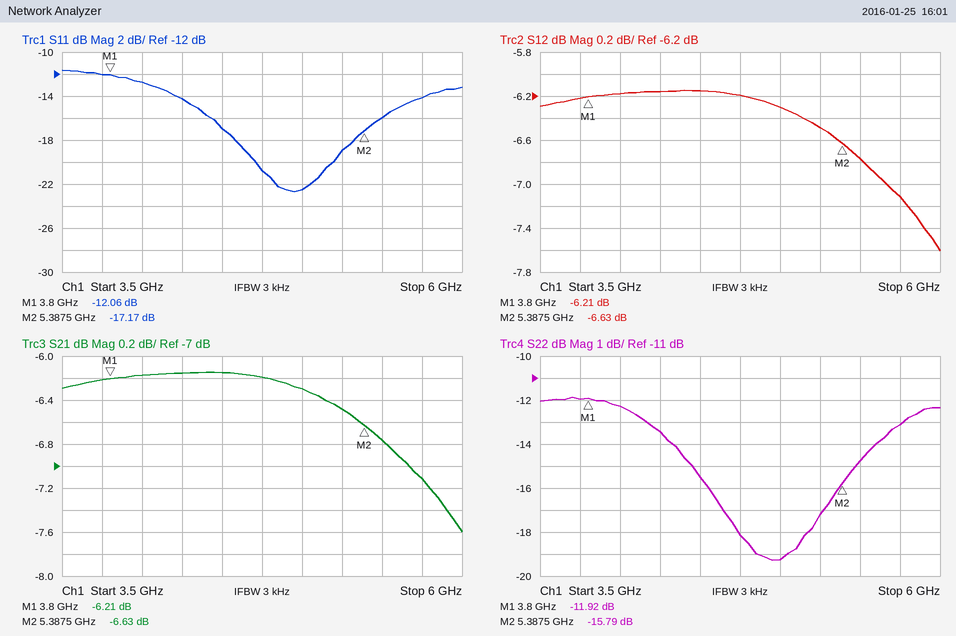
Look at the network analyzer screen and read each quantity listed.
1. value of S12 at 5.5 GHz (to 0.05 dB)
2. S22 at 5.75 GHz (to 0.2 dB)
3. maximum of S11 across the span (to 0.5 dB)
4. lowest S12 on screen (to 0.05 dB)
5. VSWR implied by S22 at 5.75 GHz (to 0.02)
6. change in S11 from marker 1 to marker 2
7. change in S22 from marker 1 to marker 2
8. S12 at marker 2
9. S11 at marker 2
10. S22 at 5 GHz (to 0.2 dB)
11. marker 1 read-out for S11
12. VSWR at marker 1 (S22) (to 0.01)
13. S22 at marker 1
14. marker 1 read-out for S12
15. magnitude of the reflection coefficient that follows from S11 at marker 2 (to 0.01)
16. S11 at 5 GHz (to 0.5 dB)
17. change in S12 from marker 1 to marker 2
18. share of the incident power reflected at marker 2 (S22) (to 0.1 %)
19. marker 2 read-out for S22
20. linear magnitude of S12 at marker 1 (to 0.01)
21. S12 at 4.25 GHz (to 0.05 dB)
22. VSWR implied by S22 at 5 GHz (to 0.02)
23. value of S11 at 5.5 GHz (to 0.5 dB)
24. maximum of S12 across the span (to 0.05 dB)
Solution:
-6.75 dB
-13.2 dB
-11.5 dB
-7.60 dB
1.56
-5.11 dB
-3.87 dB
-6.63 dB
-17.17 dB
-19.2 dB
-12.06 dB
1.68
-11.92 dB
-6.21 dB
0.14
-22.5 dB
-0.42 dB
2.6 %
-15.79 dB
0.49
-6.15 dB
1.24
-16.0 dB
-6.15 dB
